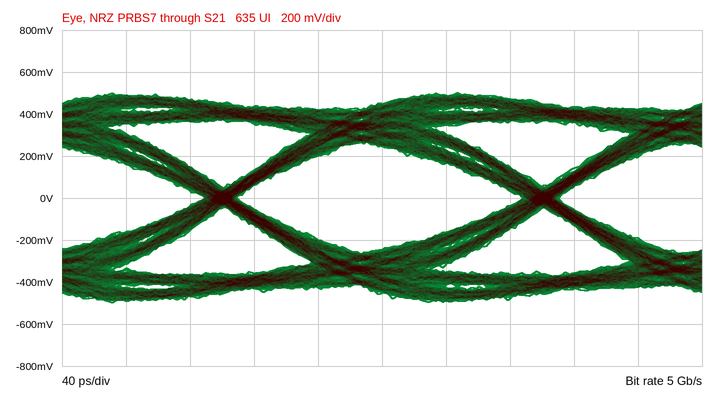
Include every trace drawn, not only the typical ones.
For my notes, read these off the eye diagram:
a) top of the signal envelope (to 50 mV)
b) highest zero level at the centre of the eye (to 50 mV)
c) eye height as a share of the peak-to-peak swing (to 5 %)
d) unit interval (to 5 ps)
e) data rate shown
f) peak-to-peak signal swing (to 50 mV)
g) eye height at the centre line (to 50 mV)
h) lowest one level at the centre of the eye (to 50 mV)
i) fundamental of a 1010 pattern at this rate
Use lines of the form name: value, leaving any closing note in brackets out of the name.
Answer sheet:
top of the signal envelope: 500 mV
highest zero level at the centre of the eye: -250 mV
eye height as a share of the peak-to-peak swing: 50 %
unit interval: 200 ps
data rate shown: 5 Gb/s
peak-to-peak signal swing: 1.00 V
eye height at the centre line: 500 mV
lowest one level at the centre of the eye: 250 mV
fundamental of a 1010 pattern at this rate: 2.5 GHz
